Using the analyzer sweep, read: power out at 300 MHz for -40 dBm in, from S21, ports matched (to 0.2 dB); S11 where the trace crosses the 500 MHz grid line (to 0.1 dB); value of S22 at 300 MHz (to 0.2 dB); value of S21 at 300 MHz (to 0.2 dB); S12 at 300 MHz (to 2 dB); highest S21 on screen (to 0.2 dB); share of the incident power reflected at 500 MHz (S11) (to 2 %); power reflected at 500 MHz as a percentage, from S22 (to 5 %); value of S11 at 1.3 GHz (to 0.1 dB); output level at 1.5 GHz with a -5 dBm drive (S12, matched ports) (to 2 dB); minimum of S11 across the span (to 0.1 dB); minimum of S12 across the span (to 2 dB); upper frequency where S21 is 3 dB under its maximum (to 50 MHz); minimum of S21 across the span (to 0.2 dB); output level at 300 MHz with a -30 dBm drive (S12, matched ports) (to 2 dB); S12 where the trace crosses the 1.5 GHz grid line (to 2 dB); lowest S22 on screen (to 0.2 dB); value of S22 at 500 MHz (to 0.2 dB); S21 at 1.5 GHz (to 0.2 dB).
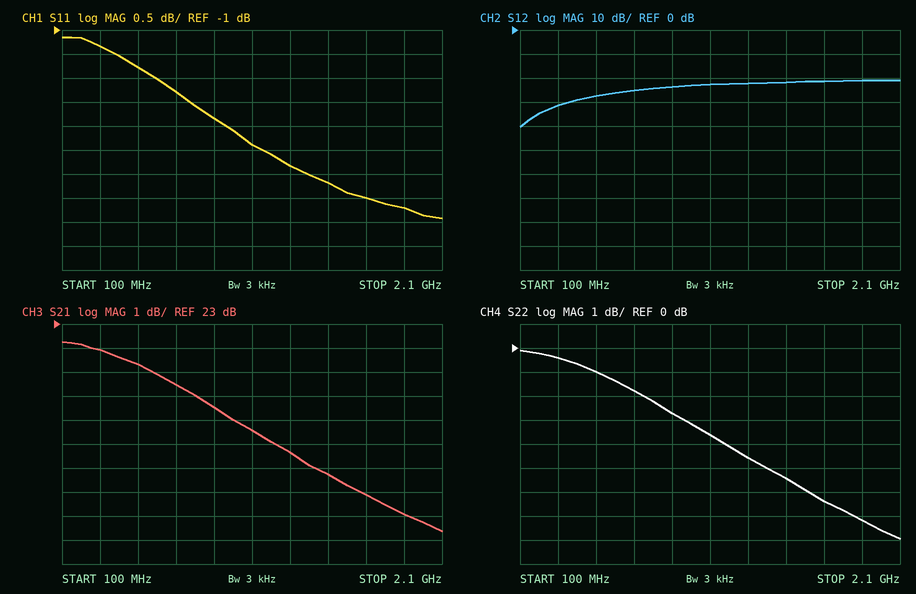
-18.0 dBm
-1.8 dB
-0.4 dB
22.0 dB
-32 dB
22.2 dB
66 %
80 %
-3.8 dB
-26 dBm
-4.9 dB
-40 dB
950 MHz
14.4 dB
-62 dBm
-22 dB
-8.0 dB
-1.0 dB
16.8 dB
